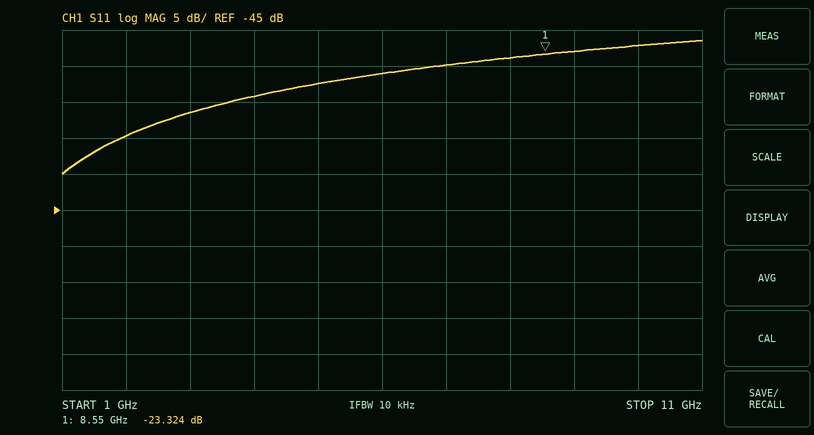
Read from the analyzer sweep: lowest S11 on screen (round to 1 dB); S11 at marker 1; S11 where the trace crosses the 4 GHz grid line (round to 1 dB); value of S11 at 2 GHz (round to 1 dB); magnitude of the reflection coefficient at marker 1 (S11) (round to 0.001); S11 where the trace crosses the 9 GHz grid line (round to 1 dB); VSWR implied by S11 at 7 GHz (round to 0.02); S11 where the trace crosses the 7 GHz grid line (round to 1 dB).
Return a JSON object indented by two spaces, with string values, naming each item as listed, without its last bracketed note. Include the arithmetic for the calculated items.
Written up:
{
  "lowest S11 on screen": "-40 dB",
  "S11 at marker 1": "-23.324 dB",
  "S11 where the trace crosses the 4 GHz grid line": "-29 dB",
  "value of S11 at 2 GHz": "-35 dB",
  "magnitude of the reflection coefficient at marker 1 (S11)": "10^(-23.324/20) ≈ 0.068",
  "S11 where the trace crosses the 9 GHz grid line": "-23 dB",
  "VSWR implied by S11 at 7 GHz": "|Γ| = 10^(-25/20) = 0.0562; VSWR = (1 + 0.0562)/(1 − 0.0562) ≈ 1.12",
  "S11 where the trace crosses the 7 GHz grid line": "-25 dB"
}
